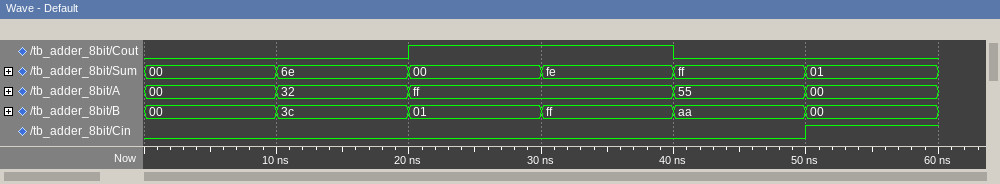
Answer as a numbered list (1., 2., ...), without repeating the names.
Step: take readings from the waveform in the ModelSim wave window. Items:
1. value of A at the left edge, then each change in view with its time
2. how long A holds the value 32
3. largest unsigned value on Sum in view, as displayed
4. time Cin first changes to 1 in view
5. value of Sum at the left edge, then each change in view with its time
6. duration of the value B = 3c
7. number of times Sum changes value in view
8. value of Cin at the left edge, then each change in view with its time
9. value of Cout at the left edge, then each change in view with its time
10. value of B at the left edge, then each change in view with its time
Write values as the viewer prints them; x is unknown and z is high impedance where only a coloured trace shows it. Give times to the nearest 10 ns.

1. 00, 32 at 10 ns, ff at 20 ns, 55 at 40 ns, 00 at 50 ns
2. 10 ns
3. ff
4. 50 ns
5. 00, 6e at 10 ns, 00 at 20 ns, fe at 30 ns, ff at 40 ns, 01 at 50 ns
6. 10 ns
7. 5
8. 0, 1 at 50 ns
9. 0, 1 at 20 ns, 0 at 40 ns
10. 00, 3c at 10 ns, 01 at 20 ns, ff at 30 ns, aa at 40 ns, 00 at 50 ns
